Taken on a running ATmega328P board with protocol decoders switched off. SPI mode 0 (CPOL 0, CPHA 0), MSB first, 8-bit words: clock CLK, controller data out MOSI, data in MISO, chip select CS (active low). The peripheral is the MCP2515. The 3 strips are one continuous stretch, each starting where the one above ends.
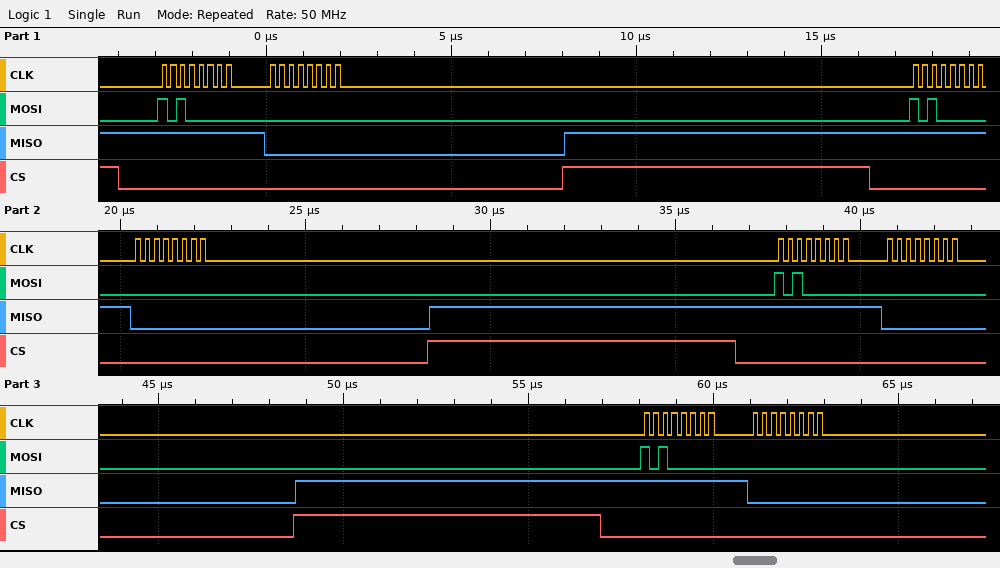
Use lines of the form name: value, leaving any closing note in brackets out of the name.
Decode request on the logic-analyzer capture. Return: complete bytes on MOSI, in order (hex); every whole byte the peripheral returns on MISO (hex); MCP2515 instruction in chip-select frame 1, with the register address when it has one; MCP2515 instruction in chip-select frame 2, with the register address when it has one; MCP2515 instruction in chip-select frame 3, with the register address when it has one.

complete bytes on MOSI, in order: 0xA0 0x00 0xA0 0x00 0xA0 0x00 0xA0 0x00
every whole byte the peripheral returns on MISO: 0xFF 0x00 0xFF 0x00 0xFF 0x00 0xFF 0x00
MCP2515 instruction in chip-select frame 1, with the register address when it has one: READ STATUS
MCP2515 instruction in chip-select frame 2, with the register address when it has one: READ STATUS
MCP2515 instruction in chip-select frame 3, with the register address when it has one: READ STATUS
